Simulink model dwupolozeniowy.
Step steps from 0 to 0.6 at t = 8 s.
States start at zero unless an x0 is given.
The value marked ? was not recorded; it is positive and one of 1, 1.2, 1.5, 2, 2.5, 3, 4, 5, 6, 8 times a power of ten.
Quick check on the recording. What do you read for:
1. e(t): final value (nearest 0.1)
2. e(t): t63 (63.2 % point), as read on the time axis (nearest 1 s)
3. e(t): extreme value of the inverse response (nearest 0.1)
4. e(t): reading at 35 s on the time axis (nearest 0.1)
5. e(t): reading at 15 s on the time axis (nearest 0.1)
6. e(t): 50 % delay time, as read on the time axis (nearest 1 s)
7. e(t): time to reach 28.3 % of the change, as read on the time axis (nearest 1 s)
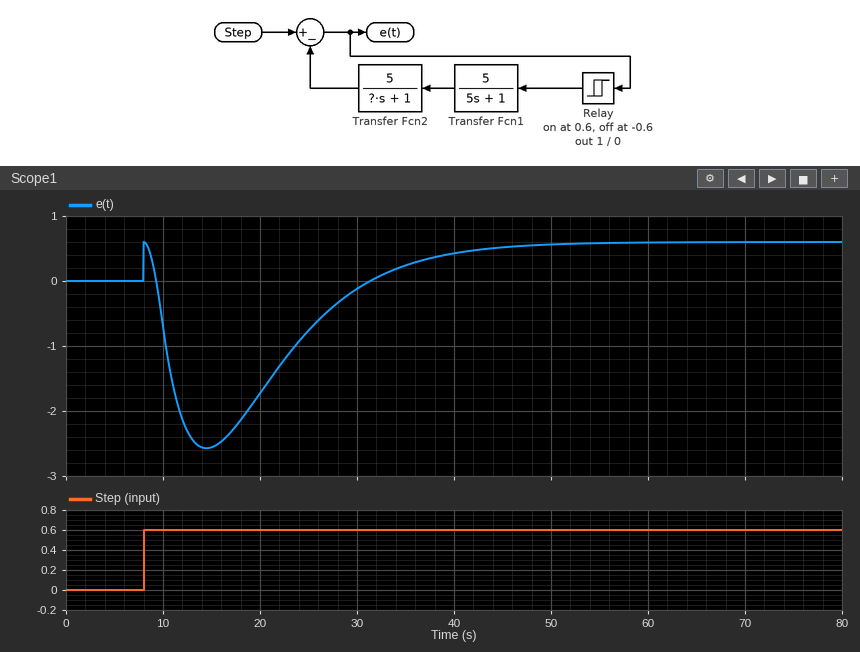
0.6
8 s
-2.6
0.2
-2.6
8 s
8 s
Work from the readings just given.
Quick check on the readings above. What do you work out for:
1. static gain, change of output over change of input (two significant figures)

1.0
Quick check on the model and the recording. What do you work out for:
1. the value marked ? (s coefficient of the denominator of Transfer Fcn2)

6
